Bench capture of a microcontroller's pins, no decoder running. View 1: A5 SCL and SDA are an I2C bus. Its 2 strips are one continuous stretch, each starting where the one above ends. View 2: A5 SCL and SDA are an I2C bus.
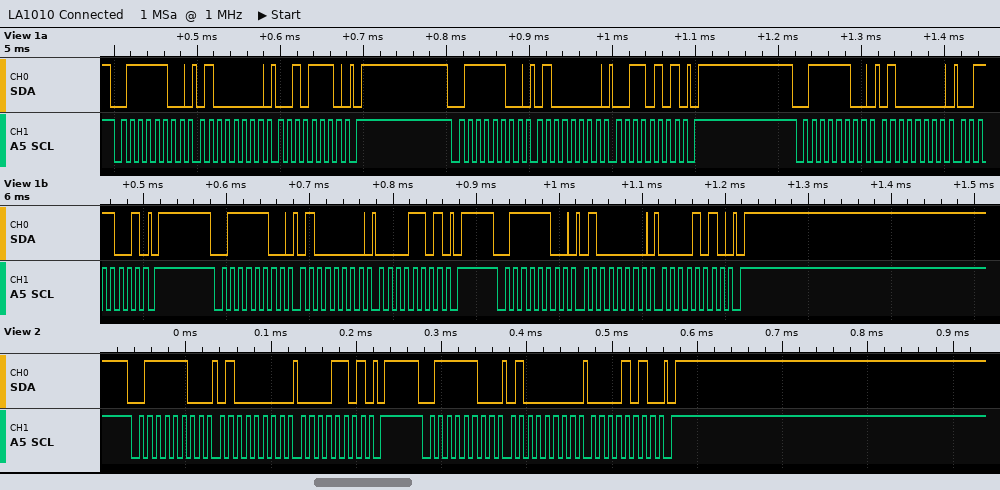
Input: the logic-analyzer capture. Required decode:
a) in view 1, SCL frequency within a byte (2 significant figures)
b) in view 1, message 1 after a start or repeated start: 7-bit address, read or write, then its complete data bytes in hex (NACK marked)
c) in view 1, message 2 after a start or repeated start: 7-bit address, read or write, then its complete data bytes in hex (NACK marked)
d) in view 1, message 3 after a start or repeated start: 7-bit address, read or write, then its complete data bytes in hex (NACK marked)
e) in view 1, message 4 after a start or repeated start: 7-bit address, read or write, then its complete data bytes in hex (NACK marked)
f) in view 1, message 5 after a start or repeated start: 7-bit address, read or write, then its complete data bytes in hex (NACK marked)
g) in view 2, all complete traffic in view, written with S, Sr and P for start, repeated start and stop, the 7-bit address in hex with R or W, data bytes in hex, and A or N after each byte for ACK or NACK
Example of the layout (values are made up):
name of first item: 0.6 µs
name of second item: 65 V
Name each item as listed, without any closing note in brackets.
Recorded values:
in view 1, SCL frequency within a byte: 100 kHz
in view 1, message 1 after a start or repeated start: 7-bit address, read or write, then its complete data bytes in hex: 0x3E write: 40 2E
in view 1, message 2 after a start or repeated start: 7-bit address, read or write, then its complete data bytes in hex: 0x3E write: 40 35
in view 1, message 3 after a start or repeated start: 7-bit address, read or write, then its complete data bytes in hex: 0x3E write: 40 39
in view 1, message 4 after a start or repeated start: 7-bit address, read or write, then its complete data bytes in hex: 0x3E write: 40 0D
in view 1, message 5 after a start or repeated start: 7-bit address, read or write, then its complete data bytes in hex: 0x3E write: 40 0A
in view 2, all complete traffic in view, written with S, Sr and P for start, repeated start and stop, the 7-bit address in hex with R or W, data bytes in hex, and A or N after each byte for ACK or NACK: S 3EW A 40 A 0D A P S 3EW A 40 A 0A A P
